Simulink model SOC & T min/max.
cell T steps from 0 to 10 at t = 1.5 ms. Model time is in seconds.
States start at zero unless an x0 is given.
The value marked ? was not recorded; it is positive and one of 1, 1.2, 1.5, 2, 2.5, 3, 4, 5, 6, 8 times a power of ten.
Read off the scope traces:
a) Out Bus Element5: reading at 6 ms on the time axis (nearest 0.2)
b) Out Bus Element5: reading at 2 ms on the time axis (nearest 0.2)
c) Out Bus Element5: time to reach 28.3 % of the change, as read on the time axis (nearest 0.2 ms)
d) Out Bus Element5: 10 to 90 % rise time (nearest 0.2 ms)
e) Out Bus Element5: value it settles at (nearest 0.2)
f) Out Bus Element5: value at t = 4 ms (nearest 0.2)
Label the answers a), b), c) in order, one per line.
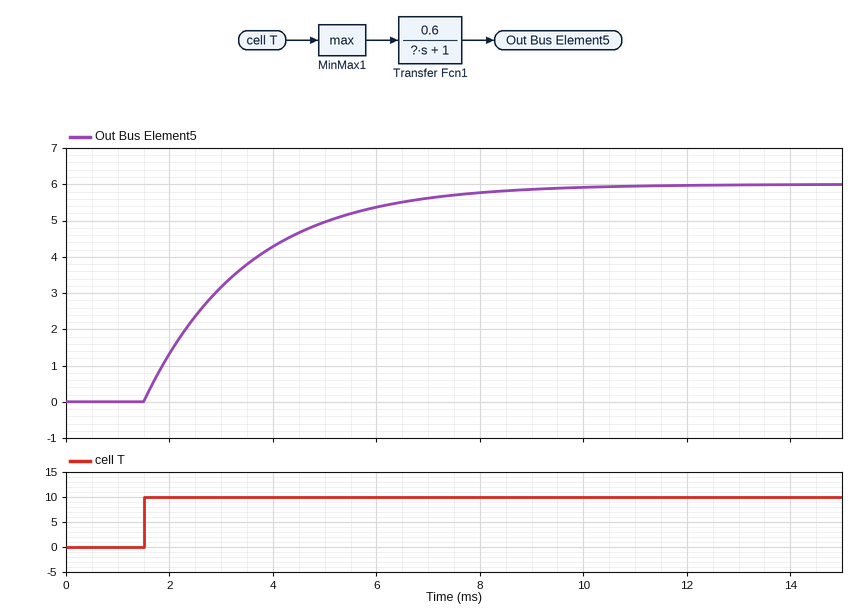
a) 5.4
b) 1.4
c) 2.2 ms
d) 4.4 ms
e) 6.0
f) 4.2
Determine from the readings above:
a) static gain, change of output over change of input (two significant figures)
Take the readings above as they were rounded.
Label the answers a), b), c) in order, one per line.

a) 0.60
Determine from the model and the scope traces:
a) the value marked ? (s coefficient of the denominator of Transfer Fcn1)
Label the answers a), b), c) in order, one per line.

a) 0.002
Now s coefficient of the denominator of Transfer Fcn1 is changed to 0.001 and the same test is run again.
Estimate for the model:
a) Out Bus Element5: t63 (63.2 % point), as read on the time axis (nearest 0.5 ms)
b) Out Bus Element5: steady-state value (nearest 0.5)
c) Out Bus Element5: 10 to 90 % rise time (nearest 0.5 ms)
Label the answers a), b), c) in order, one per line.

a) 2.5 ms
b) 6.0
c) 2.0 ms
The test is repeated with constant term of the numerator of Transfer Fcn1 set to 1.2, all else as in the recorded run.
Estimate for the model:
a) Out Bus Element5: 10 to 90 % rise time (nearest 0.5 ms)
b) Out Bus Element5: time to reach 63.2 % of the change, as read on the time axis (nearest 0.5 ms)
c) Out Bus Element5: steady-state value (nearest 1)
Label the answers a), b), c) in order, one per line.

a) 4.5 ms
b) 3.5 ms
c) 12
